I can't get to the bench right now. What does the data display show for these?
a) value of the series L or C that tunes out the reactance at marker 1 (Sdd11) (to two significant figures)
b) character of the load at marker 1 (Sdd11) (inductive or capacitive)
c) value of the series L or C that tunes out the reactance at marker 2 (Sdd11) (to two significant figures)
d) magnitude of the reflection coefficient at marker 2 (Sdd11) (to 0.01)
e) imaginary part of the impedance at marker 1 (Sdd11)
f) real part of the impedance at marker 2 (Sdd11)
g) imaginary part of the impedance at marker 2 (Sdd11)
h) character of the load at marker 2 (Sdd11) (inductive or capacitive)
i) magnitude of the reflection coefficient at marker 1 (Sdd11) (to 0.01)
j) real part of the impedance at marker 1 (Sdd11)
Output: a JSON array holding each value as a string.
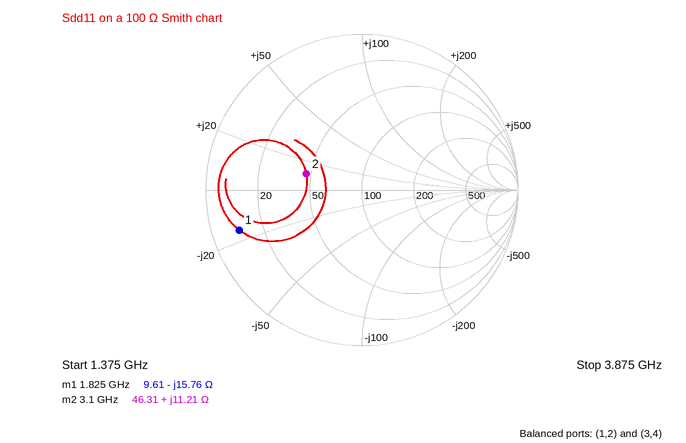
["1.4 nH", "capacitive", "4.6 pF", "0.37", "-15.76 Ω", "46.31 Ω", "+11.21 Ω", "inductive", "0.83", "9.61 Ω"]
